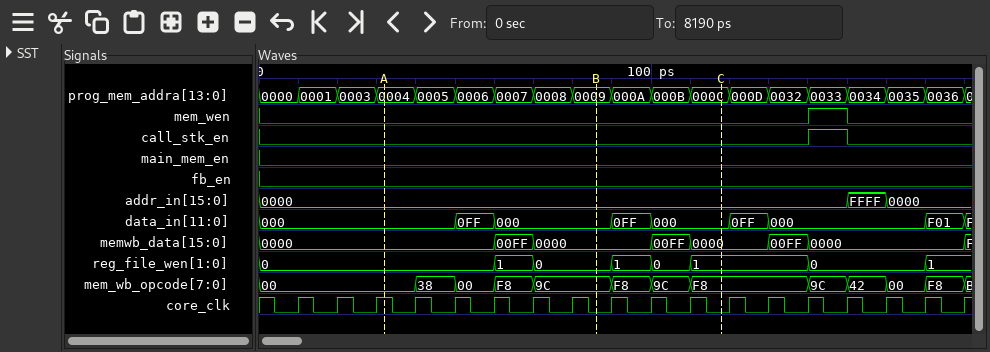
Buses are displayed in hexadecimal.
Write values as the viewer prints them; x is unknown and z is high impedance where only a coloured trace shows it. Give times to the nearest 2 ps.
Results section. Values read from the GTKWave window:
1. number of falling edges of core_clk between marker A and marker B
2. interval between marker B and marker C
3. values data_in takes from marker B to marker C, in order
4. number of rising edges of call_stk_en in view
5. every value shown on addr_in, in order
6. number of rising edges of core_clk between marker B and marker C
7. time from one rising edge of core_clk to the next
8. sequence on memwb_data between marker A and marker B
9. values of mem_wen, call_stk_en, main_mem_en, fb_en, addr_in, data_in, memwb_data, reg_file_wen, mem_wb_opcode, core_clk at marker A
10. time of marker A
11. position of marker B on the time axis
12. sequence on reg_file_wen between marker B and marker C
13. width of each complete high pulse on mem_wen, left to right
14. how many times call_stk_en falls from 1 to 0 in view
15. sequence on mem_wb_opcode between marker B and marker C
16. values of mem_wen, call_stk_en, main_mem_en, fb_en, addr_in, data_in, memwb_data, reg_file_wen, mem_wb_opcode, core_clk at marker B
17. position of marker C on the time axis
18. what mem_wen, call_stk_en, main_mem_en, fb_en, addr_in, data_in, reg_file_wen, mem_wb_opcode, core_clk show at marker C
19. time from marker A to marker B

6
32 ps
000, 0FF, 000
1
0000, FFFF, 0000
3
10 ps
0000, 00FF, 0000
mem_wen=0, call_stk_en=0, main_mem_en=0, fb_en=0, addr_in=0000, data_in=000, memwb_data=0000, reg_file_wen=0, mem_wb_opcode=00, core_clk=1
32 ps
86 ps
0, 1, 0, 1
10 ps
1
9C, F8, 9C, F8
mem_wen=0, call_stk_en=0, main_mem_en=0, fb_en=0, addr_in=0000, data_in=000, memwb_data=0000, reg_file_wen=0, mem_wb_opcode=9C, core_clk=0
118 ps
mem_wen=0, call_stk_en=0, main_mem_en=0, fb_en=0, addr_in=0000, data_in=000, reg_file_wen=1, mem_wb_opcode=F8, core_clk=0
54 ps
